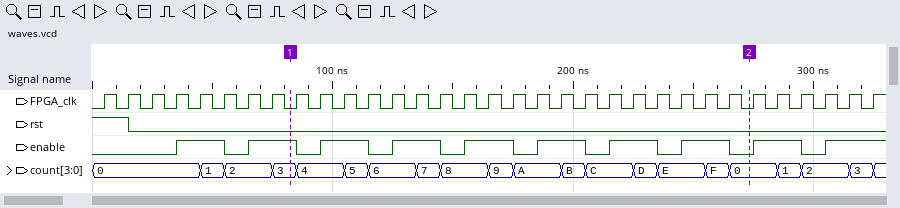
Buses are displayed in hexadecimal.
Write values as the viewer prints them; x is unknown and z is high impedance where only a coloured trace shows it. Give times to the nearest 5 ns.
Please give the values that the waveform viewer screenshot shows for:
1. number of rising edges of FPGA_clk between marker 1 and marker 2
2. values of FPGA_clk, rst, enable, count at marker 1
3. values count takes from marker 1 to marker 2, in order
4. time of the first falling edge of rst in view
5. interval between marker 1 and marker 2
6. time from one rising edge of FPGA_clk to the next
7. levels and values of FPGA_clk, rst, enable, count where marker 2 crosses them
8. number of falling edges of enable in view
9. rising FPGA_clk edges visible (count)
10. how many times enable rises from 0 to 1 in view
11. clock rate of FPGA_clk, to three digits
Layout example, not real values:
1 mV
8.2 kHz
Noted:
19
FPGA_clk=0, rst=0, enable=1, count=3
3, 4, 5, 6, 7, 8, 9, A, B, C, D, E, F, 0
15 ns
190 ns
10 ns
FPGA_clk=0, rst=0, enable=0, count=0
9
33
10
100 MHz
